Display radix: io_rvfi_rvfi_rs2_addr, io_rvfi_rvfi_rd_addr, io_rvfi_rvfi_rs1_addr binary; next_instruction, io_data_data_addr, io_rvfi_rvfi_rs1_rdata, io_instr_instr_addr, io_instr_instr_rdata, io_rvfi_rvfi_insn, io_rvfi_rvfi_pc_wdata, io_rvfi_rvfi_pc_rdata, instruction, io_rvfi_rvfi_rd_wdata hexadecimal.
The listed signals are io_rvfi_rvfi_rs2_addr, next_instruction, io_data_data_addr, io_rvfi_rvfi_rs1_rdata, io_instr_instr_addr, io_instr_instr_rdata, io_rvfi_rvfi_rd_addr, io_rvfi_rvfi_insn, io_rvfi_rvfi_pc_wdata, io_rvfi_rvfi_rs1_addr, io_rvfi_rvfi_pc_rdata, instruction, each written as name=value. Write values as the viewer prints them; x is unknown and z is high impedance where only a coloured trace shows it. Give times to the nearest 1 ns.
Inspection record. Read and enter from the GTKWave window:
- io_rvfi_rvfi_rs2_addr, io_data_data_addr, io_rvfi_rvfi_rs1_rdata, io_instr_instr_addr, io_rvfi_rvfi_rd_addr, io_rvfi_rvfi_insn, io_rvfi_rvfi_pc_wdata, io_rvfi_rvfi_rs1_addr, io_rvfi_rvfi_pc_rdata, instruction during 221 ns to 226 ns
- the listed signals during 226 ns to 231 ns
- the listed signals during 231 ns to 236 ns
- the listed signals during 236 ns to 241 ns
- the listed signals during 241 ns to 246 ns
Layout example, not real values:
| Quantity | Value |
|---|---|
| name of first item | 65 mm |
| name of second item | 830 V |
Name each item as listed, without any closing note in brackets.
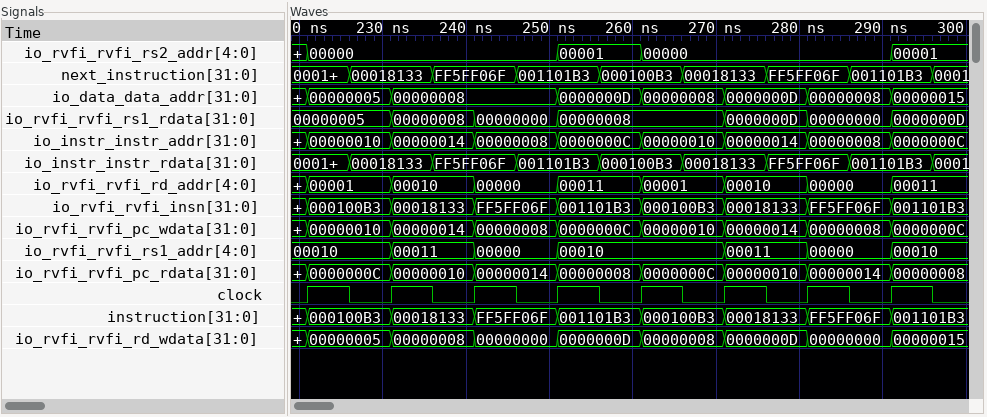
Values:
| Quantity | Value |
|---|---|
| io_rvfi_rvfi_rs2_addr, io_data_data_addr, io_rvfi_rvfi_rs1_rdata, io_instr_instr_addr, io_rvfi_rvfi_rd_addr, io_rvfi_rvfi_insn, io_rvfi_rvfi_pc_wdata, io_rvfi_rvfi_rs1_addr, io_rvfi_rvfi_pc_rdata, instruction during 221 ns to 226 ns | io_rvfi_rvfi_rs2_addr=00000, io_data_data_addr=00000005, io_rvfi_rvfi_rs1_rdata=00000005, io_instr_instr_addr=00000010, io_rvfi_rvfi_rd_addr=00001, io_rvfi_rvfi_insn=000100B3, io_rvfi_rvfi_pc_wdata=00000010, io_rvfi_rvfi_rs1_addr=00010, io_rvfi_rvfi_pc_rdata=0000000C, instruction=000100B3 |
| the listed signals during 226 ns to 231 ns | io_rvfi_rvfi_rs2_addr=00000, next_instruction=00018133, io_data_data_addr=00000005, io_rvfi_rvfi_rs1_rdata=00000005, io_instr_instr_addr=00000010, io_instr_instr_rdata=00018133, io_rvfi_rvfi_rd_addr=00001, io_rvfi_rvfi_insn=000100B3, io_rvfi_rvfi_pc_wdata=00000010, io_rvfi_rvfi_rs1_addr=00010, io_rvfi_rvfi_pc_rdata=0000000C, instruction=000100B3 |
| the listed signals during 231 ns to 236 ns | io_rvfi_rvfi_rs2_addr=00000, next_instruction=00018133, io_data_data_addr=00000008, io_rvfi_rvfi_rs1_rdata=00000008, io_instr_instr_addr=00000014, io_instr_instr_rdata=00018133, io_rvfi_rvfi_rd_addr=00010, io_rvfi_rvfi_insn=00018133, io_rvfi_rvfi_pc_wdata=00000014, io_rvfi_rvfi_rs1_addr=00011, io_rvfi_rvfi_pc_rdata=00000010, instruction=00018133 |
| the listed signals during 236 ns to 241 ns | io_rvfi_rvfi_rs2_addr=00000, next_instruction=FF5FF06F, io_data_data_addr=00000008, io_rvfi_rvfi_rs1_rdata=00000008, io_instr_instr_addr=00000014, io_instr_instr_rdata=FF5FF06F, io_rvfi_rvfi_rd_addr=00010, io_rvfi_rvfi_insn=00018133, io_rvfi_rvfi_pc_wdata=00000014, io_rvfi_rvfi_rs1_addr=00011, io_rvfi_rvfi_pc_rdata=00000010, instruction=00018133 |
| the listed signals during 241 ns to 246 ns | io_rvfi_rvfi_rs2_addr=00000, next_instruction=FF5FF06F, io_data_data_addr=00000008, io_rvfi_rvfi_rs1_rdata=00000000, io_instr_instr_addr=00000008, io_instr_instr_rdata=FF5FF06F, io_rvfi_rvfi_rd_addr=00000, io_rvfi_rvfi_insn=FF5FF06F, io_rvfi_rvfi_pc_wdata=00000008, io_rvfi_rvfi_rs1_addr=00000, io_rvfi_rvfi_pc_rdata=00000014, instruction=FF5FF06F |
